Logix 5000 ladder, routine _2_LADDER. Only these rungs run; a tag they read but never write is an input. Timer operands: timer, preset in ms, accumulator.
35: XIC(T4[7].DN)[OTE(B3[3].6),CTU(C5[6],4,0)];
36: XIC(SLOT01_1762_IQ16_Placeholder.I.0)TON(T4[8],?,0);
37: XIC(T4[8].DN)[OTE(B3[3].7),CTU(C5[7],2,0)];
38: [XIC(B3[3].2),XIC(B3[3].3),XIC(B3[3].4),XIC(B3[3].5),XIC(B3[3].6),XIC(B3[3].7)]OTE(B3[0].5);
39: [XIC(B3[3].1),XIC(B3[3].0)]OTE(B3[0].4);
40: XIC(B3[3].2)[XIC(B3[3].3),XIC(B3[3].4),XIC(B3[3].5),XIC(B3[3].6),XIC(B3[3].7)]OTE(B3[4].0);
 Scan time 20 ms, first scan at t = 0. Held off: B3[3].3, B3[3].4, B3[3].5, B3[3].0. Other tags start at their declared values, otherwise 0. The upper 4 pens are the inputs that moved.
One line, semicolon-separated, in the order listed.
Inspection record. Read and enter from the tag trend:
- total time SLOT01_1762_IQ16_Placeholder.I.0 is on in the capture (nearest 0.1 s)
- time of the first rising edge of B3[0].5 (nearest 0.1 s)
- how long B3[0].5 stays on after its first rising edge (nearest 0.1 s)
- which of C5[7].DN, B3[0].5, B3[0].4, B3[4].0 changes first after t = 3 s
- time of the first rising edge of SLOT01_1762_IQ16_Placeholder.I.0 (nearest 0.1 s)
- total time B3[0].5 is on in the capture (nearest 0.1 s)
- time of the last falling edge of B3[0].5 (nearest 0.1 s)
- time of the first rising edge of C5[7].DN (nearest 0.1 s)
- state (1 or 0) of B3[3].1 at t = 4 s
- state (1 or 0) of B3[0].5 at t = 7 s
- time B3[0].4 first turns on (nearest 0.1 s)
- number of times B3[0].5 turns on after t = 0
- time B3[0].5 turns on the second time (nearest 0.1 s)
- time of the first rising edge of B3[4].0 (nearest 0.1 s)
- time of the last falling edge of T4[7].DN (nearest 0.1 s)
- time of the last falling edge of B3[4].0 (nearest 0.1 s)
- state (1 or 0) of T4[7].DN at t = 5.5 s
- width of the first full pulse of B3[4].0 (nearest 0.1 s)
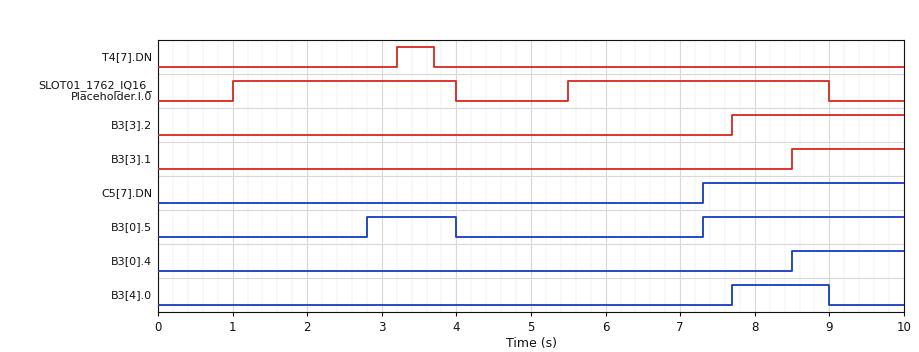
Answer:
6.5 s; 2.8 s; 1.2 s; B3[0].5; 1.0 s; 3.9 s; 4.0 s; 7.3 s; 0; 0; 8.5 s; 2; 7.3 s; 7.7 s; 3.7 s; 9.0 s; 0; 1.3 s
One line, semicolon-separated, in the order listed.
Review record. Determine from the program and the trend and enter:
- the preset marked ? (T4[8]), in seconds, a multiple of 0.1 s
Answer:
1.8 s
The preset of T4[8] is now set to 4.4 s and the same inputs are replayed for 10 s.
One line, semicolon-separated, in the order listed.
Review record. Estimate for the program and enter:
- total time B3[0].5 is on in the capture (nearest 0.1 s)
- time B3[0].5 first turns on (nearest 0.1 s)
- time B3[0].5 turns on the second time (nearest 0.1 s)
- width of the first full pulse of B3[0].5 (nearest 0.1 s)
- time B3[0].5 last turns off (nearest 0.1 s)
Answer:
2.8 s; 3.2 s; 7.7 s; 0.5 s; 3.7 s
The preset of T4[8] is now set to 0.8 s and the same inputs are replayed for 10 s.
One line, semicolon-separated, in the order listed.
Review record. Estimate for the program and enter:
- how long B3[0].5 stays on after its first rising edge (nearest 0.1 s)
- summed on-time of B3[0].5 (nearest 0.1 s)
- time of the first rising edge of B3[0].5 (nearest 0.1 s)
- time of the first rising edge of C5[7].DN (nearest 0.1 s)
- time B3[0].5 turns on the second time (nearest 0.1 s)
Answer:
2.2 s; 5.9 s; 1.8 s; 6.3 s; 6.3 s
